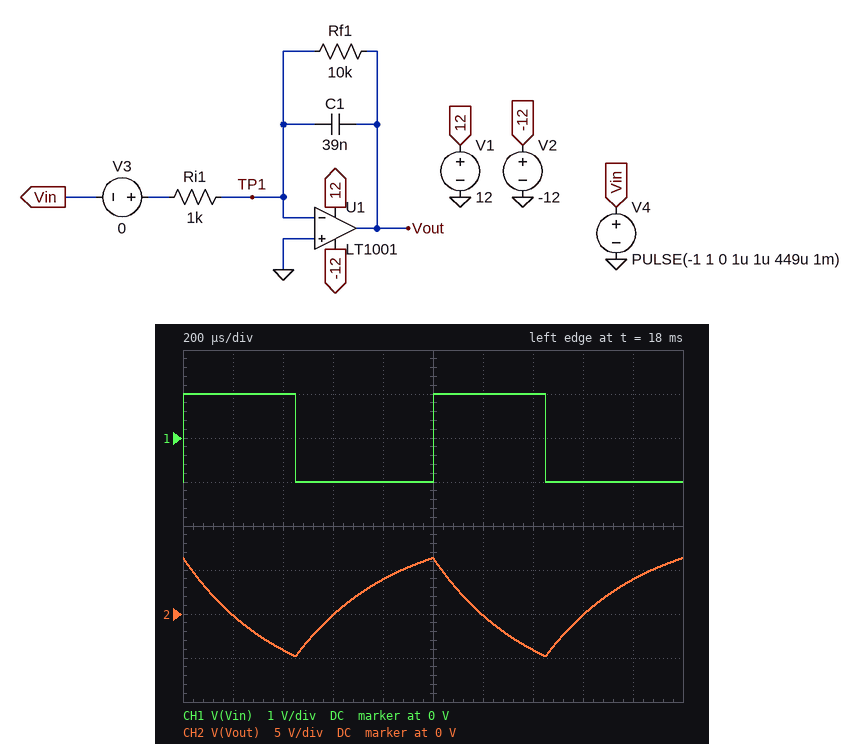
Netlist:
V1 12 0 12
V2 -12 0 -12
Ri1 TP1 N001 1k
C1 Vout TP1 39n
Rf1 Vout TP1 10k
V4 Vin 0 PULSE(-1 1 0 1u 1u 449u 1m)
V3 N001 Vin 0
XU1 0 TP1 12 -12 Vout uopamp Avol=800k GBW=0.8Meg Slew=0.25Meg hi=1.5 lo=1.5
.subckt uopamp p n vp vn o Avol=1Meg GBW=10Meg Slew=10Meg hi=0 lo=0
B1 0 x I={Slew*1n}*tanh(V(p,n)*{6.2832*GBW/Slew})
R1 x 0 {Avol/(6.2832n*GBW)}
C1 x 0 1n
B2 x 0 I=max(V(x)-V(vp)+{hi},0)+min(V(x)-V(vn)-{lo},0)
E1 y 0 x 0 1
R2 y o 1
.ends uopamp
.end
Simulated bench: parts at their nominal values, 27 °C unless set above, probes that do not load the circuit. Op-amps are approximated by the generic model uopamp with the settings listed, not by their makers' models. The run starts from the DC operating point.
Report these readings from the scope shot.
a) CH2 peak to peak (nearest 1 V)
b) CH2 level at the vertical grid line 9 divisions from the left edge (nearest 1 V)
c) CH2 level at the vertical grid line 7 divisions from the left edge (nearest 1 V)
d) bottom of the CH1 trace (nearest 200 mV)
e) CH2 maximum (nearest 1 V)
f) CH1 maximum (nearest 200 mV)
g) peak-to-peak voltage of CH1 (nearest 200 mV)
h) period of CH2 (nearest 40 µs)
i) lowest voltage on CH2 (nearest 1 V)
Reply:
11 V
4 V
-4 V
-1.0 V
6 V
1.0 V
2.0 V
1.00 ms
-5 V
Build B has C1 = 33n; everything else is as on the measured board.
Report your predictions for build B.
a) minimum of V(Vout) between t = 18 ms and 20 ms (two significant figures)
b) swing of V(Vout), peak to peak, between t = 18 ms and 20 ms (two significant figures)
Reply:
-5.6 V
13 V
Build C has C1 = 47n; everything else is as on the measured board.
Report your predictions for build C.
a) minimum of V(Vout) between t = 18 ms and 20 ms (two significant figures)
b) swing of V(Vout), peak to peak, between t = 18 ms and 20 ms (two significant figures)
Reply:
-4.0 V
9.6 V
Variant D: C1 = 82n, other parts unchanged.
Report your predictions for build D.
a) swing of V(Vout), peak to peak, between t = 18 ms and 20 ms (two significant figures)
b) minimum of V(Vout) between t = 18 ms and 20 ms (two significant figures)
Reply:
5.8 V
-2.0 V
